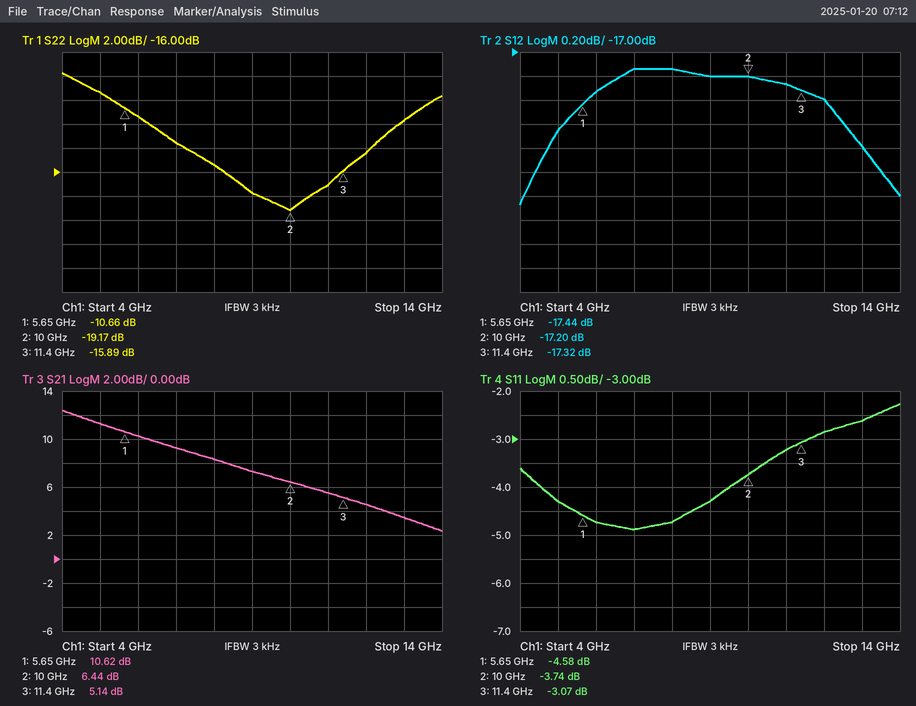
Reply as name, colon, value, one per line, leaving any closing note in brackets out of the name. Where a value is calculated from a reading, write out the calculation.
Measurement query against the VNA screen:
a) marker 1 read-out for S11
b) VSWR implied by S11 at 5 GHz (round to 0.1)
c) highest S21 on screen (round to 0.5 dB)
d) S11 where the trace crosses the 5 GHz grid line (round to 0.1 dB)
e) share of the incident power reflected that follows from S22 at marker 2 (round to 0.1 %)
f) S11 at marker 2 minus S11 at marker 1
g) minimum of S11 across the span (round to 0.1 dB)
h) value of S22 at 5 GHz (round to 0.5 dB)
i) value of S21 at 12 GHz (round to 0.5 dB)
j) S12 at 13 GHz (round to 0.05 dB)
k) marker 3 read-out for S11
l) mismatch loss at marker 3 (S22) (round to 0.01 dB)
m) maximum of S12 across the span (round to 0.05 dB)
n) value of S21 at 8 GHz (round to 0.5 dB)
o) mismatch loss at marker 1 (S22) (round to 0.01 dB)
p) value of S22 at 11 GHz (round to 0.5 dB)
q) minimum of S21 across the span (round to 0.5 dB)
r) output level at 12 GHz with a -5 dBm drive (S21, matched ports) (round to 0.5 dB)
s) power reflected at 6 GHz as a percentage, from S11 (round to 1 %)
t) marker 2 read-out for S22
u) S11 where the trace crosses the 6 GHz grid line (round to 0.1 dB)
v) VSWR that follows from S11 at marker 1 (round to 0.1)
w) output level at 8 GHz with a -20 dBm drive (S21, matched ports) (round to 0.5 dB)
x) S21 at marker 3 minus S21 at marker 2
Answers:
marker 1 read-out for S11: -4.58 dB
VSWR implied by S11 at 5 GHz: |Γ| = 10^(-4.3/20) = 0.6095; VSWR = (1 + 0.6095)/(1 − 0.6095) ≈ 4.1
highest S21 on screen: 12.5 dB
S11 where the trace crosses the 5 GHz grid line: -4.3 dB
share of the incident power reflected that follows from S22 at marker 2: 10^(-19.17/10) ≈ 1.2 %
S11 at marker 2 minus S11 at marker 1: -3.74 − (-4.58) = 0.84 dB
minimum of S11 across the span: -4.9 dB
value of S22 at 5 GHz: -9.5 dB
value of S21 at 12 GHz: 4.5 dB
S12 at 13 GHz: -17.80 dB
marker 3 read-out for S11: -3.07 dB
mismatch loss at marker 3 (S22): −10 log10(1 − 10^(-15.89/10)) ≈ 0.11 dB
maximum of S12 across the span: -17.15 dB
value of S21 at 8 GHz: 8.5 dB
mismatch loss at marker 1 (S22): −10 log10(1 − 10^(-10.66/10)) ≈ 0.39 dB
value of S22 at 11 GHz: -17.0 dB
minimum of S21 across the span: 2.5 dB
output level at 12 GHz with a -5 dBm drive (S21, matched ports): -5 dBm + (4.5 dB) = -0.5 dBm
power reflected at 6 GHz as a percentage, from S11: 10^(-4.7/10) ≈ 34 %
marker 2 read-out for S22: -19.17 dB
S11 where the trace crosses the 6 GHz grid line: -4.7 dB
VSWR that follows from S11 at marker 1: (1 + 0.5902)/(1 − 0.5902) ≈ 3.9
output level at 8 GHz with a -20 dBm drive (S21, matched ports): -20 dBm + (8.5 dB) = -11.5 dBm
S21 at marker 3 minus S21 at marker 2: 5.14 − (6.44) = -1.30 dB
